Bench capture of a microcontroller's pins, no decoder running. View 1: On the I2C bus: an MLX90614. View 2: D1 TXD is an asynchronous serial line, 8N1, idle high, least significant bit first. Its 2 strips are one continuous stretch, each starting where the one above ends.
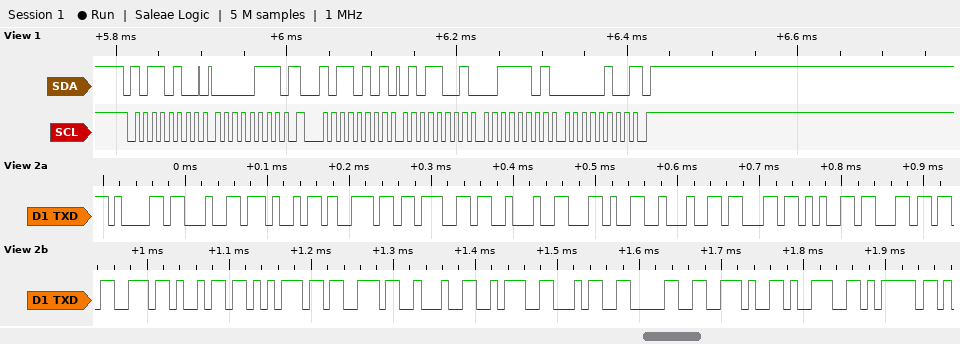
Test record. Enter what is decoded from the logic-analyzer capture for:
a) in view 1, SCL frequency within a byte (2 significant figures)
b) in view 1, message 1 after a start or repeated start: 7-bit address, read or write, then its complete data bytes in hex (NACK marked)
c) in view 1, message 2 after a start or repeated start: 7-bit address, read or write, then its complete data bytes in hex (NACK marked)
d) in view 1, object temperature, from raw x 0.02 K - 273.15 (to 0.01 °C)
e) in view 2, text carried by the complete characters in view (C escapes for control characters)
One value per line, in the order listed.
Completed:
100 kHz
0x5A write: 07
0x5A read: 59 3D 04 NACK
40.95 °C
"ading\",\"celsius\":40.9}"
